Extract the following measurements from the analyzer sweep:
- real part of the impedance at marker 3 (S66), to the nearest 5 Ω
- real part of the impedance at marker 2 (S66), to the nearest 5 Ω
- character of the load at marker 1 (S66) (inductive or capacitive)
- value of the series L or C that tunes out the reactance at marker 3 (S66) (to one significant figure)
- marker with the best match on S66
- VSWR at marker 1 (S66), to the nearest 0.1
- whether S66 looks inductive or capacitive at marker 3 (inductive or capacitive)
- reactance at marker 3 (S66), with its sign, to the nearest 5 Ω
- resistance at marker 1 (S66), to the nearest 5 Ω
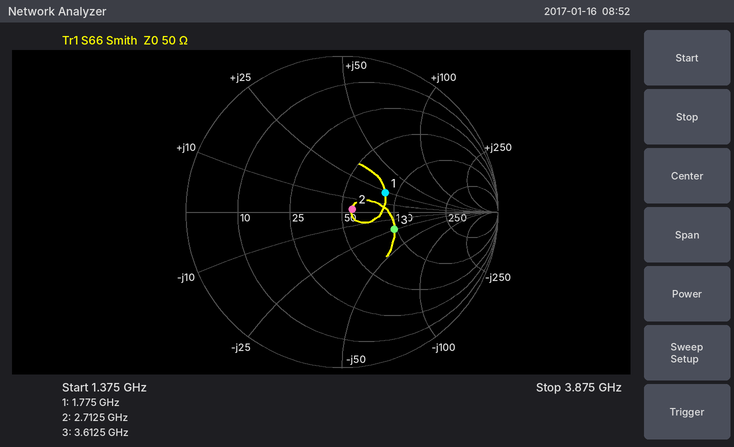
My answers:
95 Ω
55 Ω
inductive
1 nH
marker 2
1.9
capacitive
-25 Ω
85 Ω
